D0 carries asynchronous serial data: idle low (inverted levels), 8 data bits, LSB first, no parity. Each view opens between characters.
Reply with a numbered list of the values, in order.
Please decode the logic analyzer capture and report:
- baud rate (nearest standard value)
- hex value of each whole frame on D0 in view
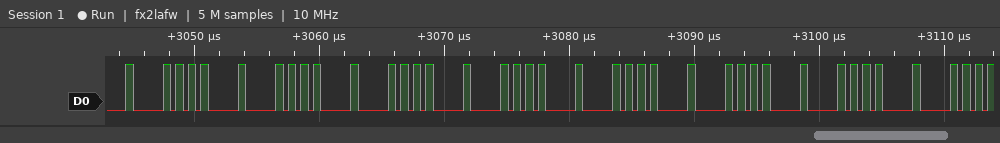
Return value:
1. 2000000 baud
2. 5F, 7D, D5, 5F, 7D, D5, 5F, 7D, D5, 5F, 7D
